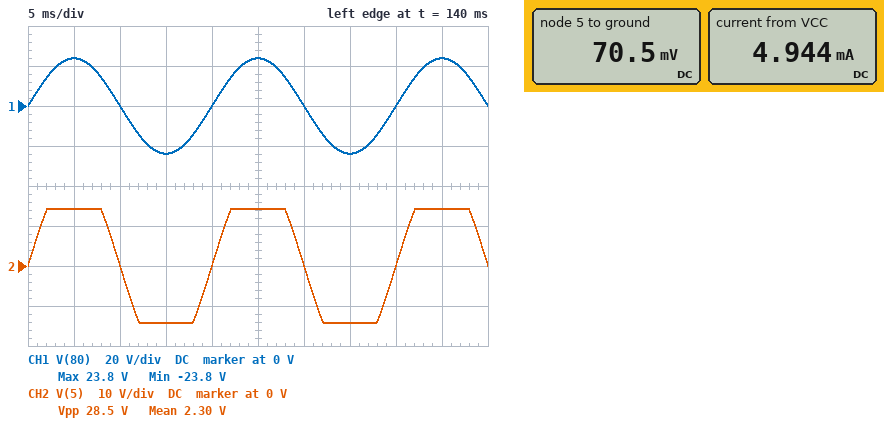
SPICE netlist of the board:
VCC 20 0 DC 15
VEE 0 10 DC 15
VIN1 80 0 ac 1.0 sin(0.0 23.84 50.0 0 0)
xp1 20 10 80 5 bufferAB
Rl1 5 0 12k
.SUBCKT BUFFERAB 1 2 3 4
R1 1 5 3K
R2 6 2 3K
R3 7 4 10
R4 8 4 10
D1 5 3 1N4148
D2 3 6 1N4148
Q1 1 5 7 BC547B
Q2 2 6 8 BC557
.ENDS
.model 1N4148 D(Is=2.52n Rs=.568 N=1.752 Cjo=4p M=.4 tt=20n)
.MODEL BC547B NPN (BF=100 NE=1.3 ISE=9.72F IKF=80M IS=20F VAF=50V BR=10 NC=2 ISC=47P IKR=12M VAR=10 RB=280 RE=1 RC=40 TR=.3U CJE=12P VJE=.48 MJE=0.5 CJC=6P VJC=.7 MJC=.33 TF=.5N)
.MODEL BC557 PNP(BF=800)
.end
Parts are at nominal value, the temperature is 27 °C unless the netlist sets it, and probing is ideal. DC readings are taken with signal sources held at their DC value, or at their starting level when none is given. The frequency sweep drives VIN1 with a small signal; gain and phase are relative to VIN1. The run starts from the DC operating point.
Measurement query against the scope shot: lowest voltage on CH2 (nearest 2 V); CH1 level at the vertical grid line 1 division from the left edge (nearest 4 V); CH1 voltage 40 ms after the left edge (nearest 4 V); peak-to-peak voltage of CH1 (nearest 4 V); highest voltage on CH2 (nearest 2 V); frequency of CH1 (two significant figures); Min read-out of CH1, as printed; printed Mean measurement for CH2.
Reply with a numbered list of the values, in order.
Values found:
1. -14 V
2. 24 V
3. 0 V
4. 48 V
5. 14 V
6. 50 Hz
7. -23.8 V
8. 2.30 V
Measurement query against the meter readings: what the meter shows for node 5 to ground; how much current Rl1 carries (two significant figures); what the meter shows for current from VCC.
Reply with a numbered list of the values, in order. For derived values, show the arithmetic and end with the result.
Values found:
1. 70.5 mV
2. (70.5 mV) / 12 kΩ = 5.9 µA
3. 4.944 mA
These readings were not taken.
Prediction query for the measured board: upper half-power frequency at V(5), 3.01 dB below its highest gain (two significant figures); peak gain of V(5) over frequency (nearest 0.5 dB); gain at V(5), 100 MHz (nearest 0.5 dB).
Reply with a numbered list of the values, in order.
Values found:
1. 560 MHz
2. 0 dB
3. -0.5 dB
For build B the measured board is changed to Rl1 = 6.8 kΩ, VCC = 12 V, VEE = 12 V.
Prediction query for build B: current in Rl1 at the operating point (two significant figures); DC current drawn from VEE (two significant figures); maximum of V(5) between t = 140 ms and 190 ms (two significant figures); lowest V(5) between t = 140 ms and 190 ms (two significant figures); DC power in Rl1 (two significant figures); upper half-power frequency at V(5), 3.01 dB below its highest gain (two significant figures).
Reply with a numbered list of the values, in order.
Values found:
1. 10 µA
2. 3.9 mA
3. 11 V
4. -11 V
5. 700 nW
6. 430 MHz
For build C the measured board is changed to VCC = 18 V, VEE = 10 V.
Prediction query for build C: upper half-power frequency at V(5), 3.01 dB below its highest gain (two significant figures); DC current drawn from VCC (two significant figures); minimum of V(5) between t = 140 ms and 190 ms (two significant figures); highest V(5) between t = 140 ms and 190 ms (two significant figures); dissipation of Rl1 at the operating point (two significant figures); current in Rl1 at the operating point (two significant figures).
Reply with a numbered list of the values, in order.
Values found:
1. 550 MHz
2. 5.9 mA
3. -9.2 V
4. 17 V
5. 610 nW
6. 7.1 µA
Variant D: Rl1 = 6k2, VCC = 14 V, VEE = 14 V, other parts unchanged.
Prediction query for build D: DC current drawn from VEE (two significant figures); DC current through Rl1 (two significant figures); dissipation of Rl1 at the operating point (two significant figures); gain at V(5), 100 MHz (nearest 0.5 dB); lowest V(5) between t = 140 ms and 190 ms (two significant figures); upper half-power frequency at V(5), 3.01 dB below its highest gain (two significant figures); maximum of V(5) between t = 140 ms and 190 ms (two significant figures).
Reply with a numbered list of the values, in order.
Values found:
1. 4.6 mA
2. 11 µA
3. 780 nW
4. -0.5 dB
5. -13 V
6. 510 MHz
7. 13 V
